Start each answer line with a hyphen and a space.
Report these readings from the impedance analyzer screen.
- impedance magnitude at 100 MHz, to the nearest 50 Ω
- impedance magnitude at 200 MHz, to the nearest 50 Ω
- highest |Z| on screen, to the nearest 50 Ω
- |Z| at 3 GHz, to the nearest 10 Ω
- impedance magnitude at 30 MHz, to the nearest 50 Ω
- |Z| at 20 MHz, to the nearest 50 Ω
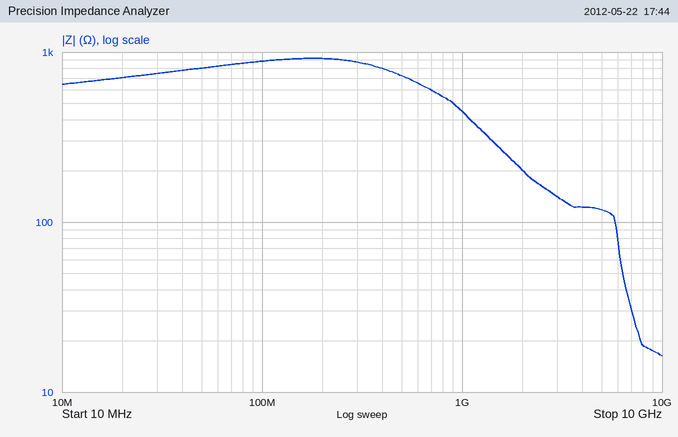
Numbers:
- 900 Ω
- 900 Ω
- 900 Ω
- 140 Ω
- 750 Ω
- 700 Ω
